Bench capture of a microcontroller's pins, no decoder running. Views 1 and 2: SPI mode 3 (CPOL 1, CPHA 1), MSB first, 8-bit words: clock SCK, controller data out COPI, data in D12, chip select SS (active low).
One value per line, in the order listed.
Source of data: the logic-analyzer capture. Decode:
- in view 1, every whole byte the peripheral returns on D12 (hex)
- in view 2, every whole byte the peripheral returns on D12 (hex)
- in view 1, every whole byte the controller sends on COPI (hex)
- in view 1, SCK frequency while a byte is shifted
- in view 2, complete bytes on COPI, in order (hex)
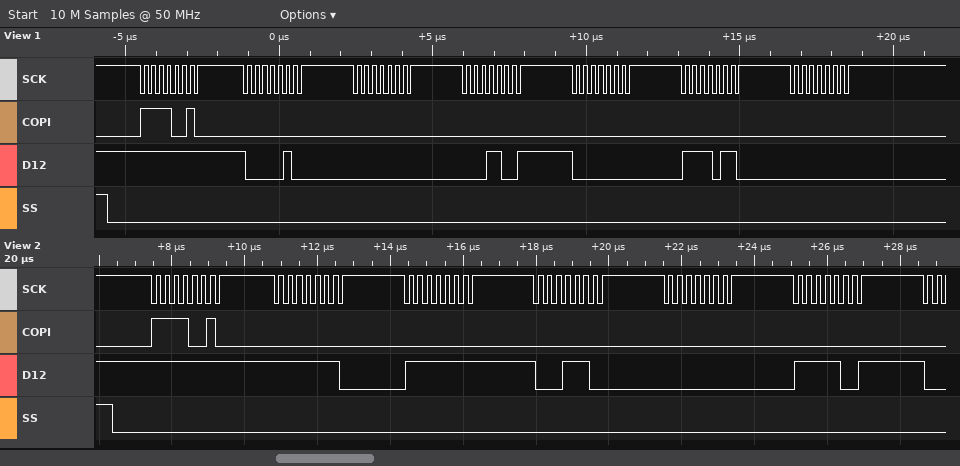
FF 04 00 19 00 F6 00
0xFF 0xFE 0xFF 0x1C 0x00 0xF9
F2 00 00 00 00 00 00
4 MHz
0xF2 0x00 0x00 0x00 0x00 0x00
